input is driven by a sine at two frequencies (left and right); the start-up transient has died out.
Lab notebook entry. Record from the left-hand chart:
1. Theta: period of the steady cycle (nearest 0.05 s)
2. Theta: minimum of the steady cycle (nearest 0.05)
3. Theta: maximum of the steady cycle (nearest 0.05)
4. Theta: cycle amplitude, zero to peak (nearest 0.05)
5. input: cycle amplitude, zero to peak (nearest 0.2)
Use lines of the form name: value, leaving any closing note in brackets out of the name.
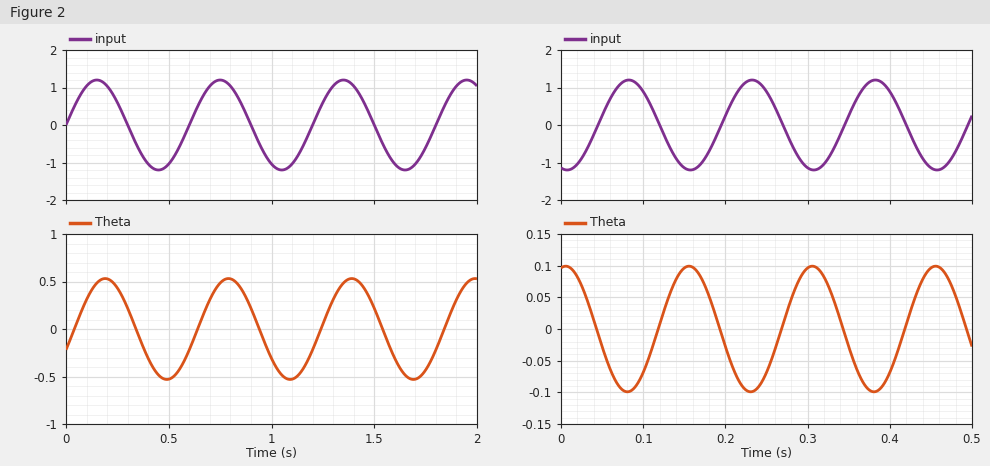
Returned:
Theta: period of the steady cycle: 0.60 s
Theta: minimum of the steady cycle: -0.55
Theta: maximum of the steady cycle: 0.55
Theta: cycle amplitude, zero to peak: 0.55
input: cycle amplitude, zero to peak: 1.2
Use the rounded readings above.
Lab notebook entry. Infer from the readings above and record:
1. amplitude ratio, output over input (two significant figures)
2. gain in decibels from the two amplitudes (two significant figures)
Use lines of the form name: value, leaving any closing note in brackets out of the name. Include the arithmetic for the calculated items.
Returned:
amplitude ratio, output over input: 0.55 / 1.2 = 0.46
gain in decibels from the two amplitudes: 20 log10(0.55 / 1.2) = -6.8 dB
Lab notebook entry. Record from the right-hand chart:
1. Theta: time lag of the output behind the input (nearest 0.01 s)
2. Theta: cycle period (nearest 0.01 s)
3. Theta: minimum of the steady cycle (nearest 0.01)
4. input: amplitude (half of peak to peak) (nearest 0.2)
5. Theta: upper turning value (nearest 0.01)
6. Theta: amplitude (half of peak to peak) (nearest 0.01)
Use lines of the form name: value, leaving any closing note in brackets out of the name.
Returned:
Theta: time lag of the output behind the input: 0.07 s
Theta: cycle period: 0.15 s
Theta: minimum of the steady cycle: -0.10
input: amplitude (half of peak to peak): 1.2
Theta: upper turning value: 0.10
Theta: amplitude (half of peak to peak): 0.10
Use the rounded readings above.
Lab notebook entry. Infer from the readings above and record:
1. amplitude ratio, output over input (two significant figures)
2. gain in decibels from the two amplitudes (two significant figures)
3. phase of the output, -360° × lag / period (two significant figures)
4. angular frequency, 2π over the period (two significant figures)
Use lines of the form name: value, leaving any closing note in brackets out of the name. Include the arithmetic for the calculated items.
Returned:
amplitude ratio, output over input: 0.1 / 1.2 = 0.083
gain in decibels from the two amplitudes: 20 log10(0.1 / 1.2) = -22 dB
phase of the output, -360° × lag / period: -360 × 0.07 / 0.15 = -170°
angular frequency, 2π over the period: 2π / 0.15 = 42 rad/s
